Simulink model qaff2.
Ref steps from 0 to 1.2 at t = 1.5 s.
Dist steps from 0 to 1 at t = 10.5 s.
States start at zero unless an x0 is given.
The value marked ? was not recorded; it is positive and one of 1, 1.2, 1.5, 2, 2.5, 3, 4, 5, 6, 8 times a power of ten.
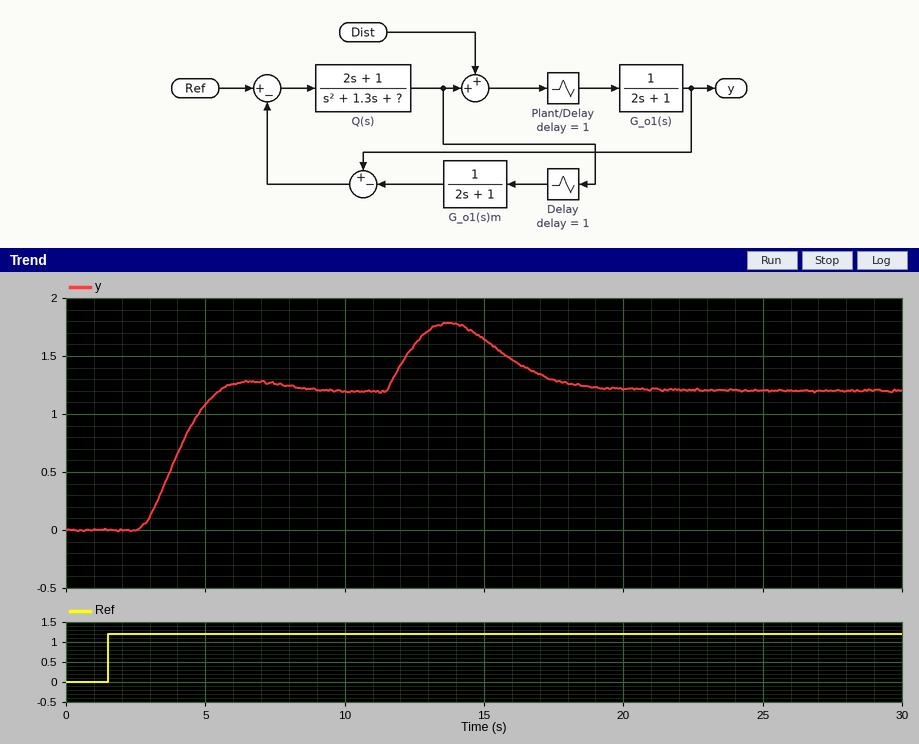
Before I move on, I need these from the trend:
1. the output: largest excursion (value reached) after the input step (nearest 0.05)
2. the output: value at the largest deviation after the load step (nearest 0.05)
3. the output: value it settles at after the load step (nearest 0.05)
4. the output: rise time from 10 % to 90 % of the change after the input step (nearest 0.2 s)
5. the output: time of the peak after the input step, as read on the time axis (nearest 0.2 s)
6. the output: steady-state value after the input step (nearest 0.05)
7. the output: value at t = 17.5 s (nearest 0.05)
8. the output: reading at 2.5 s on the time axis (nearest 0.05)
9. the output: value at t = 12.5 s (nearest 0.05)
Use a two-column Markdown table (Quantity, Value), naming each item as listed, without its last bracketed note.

| Quantity | Value |
|---|---|
| the output: largest excursion (value reached) after the input step | 1.30 |
| the output: value at the largest deviation after the load step | 1.80 |
| the output: value it settles at after the load step | 1.20 |
| the output: rise time from 10 % to 90 % of the change after the input step | 2.0 s |
| the output: time of the peak after the input step, as read on the time axis | 6.6 s |
| the output: steady-state value after the input step | 1.20 |
| the output: value at t = 17.5 s | 1.30 |
| the output: reading at 2.5 s on the time axis | 0.00 |
| the output: value at t = 12.5 s | 1.60 |
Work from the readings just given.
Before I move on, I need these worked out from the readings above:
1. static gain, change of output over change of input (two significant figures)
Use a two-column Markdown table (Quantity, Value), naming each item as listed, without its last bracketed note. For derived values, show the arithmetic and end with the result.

| Quantity | Value |
|---|---|
| static gain, change of output over change of input | (1.2 - 0) / (1.2 - 0) = 1.0 |
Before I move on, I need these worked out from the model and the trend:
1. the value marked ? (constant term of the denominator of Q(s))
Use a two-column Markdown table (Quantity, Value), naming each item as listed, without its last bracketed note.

| Quantity | Value |
|---|---|
| the value marked ? (constant term of the denominator of Q(s)) | 1 |
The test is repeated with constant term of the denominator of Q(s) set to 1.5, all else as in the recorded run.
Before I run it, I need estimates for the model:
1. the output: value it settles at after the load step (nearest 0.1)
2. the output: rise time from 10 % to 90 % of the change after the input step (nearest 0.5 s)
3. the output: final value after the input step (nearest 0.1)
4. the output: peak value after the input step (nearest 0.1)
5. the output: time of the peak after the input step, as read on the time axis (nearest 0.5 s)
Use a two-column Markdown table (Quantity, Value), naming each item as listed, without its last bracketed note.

| Quantity | Value |
|---|---|
| the output: value it settles at after the load step | 1.1 |
| the output: rise time from 10 % to 90 % of the change after the input step | 1.5 s |
| the output: final value after the input step | 0.8 |
| the output: peak value after the input step | 0.9 |
| the output: time of the peak after the input step, as read on the time axis | 5.5 s |
